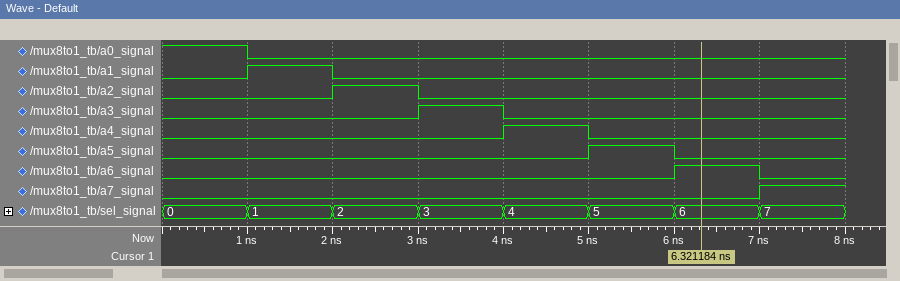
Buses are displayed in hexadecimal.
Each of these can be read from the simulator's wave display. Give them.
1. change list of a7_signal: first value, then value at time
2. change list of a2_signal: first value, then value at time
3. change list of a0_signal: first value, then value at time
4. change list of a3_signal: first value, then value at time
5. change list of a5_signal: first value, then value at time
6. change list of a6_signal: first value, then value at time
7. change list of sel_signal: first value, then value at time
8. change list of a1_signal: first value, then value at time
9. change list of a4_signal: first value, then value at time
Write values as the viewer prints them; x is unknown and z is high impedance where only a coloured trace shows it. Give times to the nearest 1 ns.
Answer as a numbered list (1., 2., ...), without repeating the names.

1. 0, 1 at 7 ns
2. 0, 1 at 2 ns, 0 at 3 ns
3. 1, 0 at 1 ns
4. 0, 1 at 3 ns, 0 at 4 ns
5. 0, 1 at 5 ns, 0 at 6 ns
6. 0, 1 at 6 ns, 0 at 7 ns
7. 0, 1 at 1 ns, 2 at 2 ns, 3 at 3 ns, 4 at 4 ns, 5 at 5 ns, 6 at 6 ns, 7 at 7 ns
8. 0, 1 at 1 ns, 0 at 2 ns
9. 0, 1 at 4 ns, 0 at 5 ns
